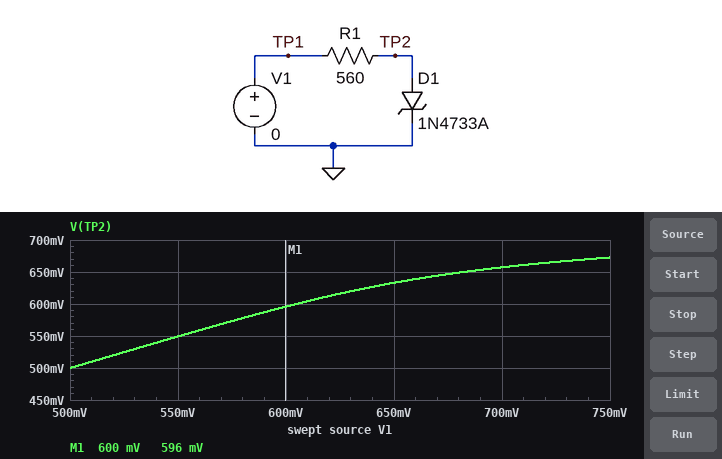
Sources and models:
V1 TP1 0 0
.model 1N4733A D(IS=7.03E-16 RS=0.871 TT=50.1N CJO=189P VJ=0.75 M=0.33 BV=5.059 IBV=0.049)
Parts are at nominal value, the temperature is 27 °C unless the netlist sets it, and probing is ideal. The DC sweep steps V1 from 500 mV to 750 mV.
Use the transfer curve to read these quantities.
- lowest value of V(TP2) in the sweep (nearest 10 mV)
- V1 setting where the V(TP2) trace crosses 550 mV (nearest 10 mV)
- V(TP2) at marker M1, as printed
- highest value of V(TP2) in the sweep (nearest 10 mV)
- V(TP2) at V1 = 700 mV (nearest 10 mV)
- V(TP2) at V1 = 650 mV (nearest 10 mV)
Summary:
500 mV
550 mV
596 mV
670 mV
660 mV
630 mV
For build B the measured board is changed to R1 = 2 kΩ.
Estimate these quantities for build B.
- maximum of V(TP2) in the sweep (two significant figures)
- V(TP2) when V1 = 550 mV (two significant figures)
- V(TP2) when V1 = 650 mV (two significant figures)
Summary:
650 mV
550 mV
620 mV
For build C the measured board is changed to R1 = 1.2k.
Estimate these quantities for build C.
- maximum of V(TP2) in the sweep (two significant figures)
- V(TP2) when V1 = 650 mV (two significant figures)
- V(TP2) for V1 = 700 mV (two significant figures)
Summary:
660 mV
620 mV
640 mV
